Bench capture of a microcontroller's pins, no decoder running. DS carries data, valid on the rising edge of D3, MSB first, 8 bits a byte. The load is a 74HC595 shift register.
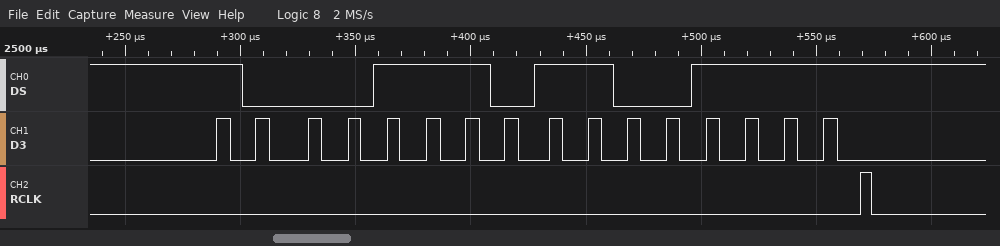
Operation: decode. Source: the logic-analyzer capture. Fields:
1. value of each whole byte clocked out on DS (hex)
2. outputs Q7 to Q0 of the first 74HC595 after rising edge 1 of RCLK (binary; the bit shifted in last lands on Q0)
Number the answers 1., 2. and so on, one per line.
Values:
1. 0x8E 0xCF
2. 11001111
